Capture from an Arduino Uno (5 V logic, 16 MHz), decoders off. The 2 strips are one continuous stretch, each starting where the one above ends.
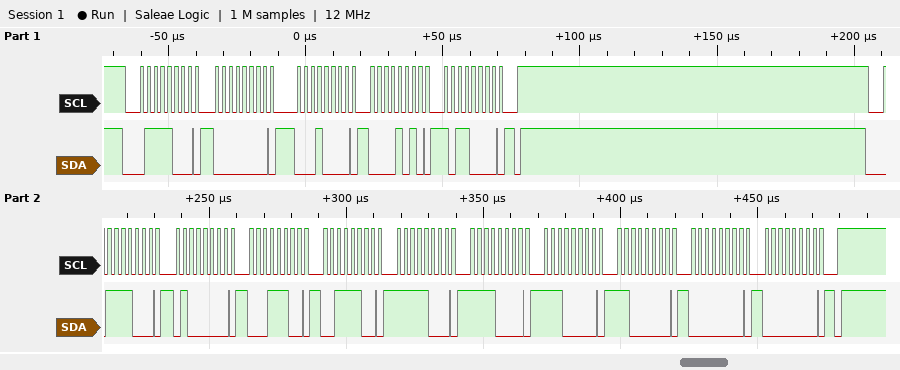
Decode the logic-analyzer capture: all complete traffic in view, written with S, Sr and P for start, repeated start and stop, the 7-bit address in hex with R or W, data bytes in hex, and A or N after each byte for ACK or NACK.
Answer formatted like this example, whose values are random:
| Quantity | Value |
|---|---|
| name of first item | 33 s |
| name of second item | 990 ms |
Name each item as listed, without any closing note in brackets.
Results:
| Quantity | Value |
|---|---|
| all complete traffic in view, written with S, Sr and P for start, repeated start and stop, the 7-bit address in hex with R or W, data bytes in hex, and A or N after each byte for ACK or NACK | S 3CW A 00 A 10 A 0A A B0 A P S 3CW A 40 A 1C A 3C A F8 A F0 A E0 A C0 A 00 A 00 A P |
